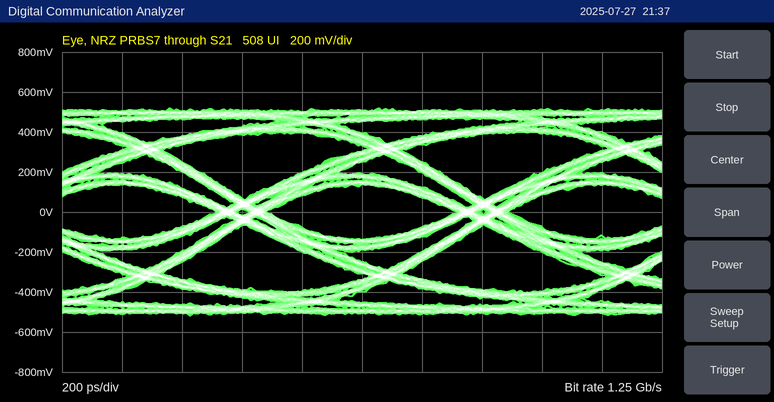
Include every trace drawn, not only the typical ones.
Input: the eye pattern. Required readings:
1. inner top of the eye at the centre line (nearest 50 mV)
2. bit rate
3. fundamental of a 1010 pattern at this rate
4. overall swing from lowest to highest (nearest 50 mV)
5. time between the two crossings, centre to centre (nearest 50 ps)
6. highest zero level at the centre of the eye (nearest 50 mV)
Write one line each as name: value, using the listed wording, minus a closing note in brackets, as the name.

inner top of the eye at the centre line: 150 mV
bit rate: 1.25 Gb/s
fundamental of a 1010 pattern at this rate: 625 MHz
overall swing from lowest to highest: 1.05 V
time between the two crossings, centre to centre: 800 ps
highest zero level at the centre of the eye: -150 mV
